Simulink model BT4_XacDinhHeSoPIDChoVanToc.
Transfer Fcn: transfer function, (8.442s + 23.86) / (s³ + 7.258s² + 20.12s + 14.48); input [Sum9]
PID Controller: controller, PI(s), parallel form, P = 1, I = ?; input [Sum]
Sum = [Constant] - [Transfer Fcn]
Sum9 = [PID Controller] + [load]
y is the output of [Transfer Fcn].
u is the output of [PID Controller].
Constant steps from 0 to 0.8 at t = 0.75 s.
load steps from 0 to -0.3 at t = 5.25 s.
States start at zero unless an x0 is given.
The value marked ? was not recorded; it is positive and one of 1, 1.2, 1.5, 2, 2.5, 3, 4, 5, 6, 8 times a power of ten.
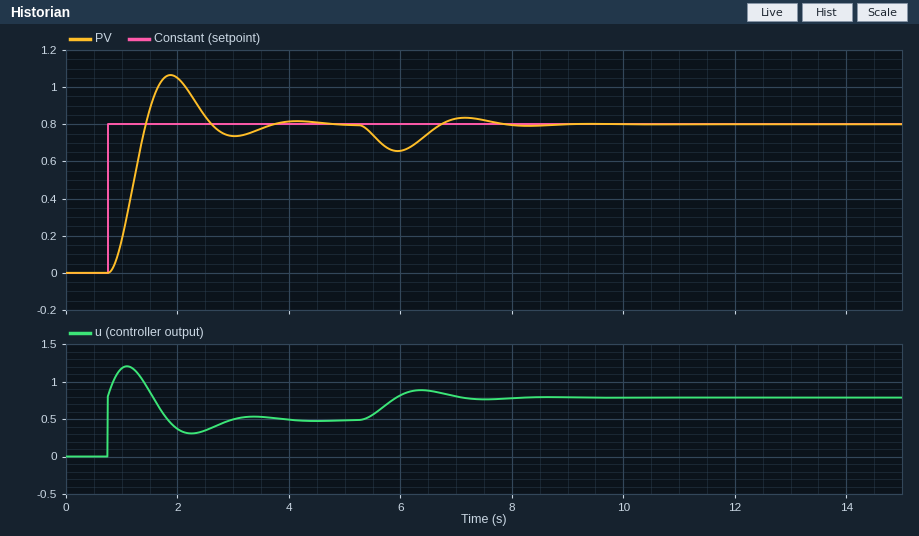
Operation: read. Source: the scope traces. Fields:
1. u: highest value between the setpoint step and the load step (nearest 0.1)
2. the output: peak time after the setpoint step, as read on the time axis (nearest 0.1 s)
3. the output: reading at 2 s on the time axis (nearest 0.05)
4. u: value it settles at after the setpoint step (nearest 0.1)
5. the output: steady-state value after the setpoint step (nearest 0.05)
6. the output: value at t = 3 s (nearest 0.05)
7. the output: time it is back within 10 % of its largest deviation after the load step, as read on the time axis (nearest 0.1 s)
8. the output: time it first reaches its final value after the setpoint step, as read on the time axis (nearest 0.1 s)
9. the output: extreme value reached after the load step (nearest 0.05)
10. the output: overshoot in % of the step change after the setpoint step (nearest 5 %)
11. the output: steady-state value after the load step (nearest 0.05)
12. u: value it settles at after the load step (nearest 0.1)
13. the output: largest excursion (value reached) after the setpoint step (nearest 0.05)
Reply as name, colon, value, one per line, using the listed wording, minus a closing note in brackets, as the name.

u: highest value between the setpoint step and the load step: 1.2
the output: peak time after the setpoint step, as read on the time axis: 1.9 s
the output: reading at 2 s on the time axis: 1.05
u: value it settles at after the setpoint step: 0.5
the output: steady-state value after the setpoint step: 0.80
the output: value at t = 3 s: 0.75
the output: time it is back within 10 % of its largest deviation after the load step, as read on the time axis: 7.6 s
the output: time it first reaches its final value after the setpoint step, as read on the time axis: 1.4 s
the output: extreme value reached after the load step: 0.65
the output: overshoot in % of the step change after the setpoint step: 35 %
the output: steady-state value after the load step: 0.80
u: value it settles at after the load step: 0.8
the output: largest excursion (value reached) after the setpoint step: 1.05
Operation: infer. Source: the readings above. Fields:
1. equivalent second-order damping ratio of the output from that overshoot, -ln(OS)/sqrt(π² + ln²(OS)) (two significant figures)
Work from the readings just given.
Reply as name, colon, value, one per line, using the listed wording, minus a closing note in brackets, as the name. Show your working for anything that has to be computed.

equivalent second-order damping ratio of the output from that overshoot, -ln(OS)/sqrt(π² + ln²(OS)): ln(0.35) = -1.050; 1.050 / sqrt(9.870 + 1.102) = 0.32
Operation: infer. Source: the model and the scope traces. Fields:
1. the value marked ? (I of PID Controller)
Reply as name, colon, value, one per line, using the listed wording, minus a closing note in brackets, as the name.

the value marked ?: 3
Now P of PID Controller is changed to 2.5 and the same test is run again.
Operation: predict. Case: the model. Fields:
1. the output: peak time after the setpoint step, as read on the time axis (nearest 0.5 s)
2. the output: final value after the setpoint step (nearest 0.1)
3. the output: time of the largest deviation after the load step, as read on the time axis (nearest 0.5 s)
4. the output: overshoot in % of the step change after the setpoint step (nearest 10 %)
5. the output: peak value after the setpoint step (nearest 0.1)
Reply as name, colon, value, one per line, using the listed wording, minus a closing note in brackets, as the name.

the output: peak time after the setpoint step, as read on the time axis: 1.5 s
the output: final value after the setpoint step: 0.8
the output: time of the largest deviation after the load step, as read on the time axis: 6.0 s
the output: overshoot in % of the step change after the setpoint step: 20 %
the output: peak value after the setpoint step: 1.0
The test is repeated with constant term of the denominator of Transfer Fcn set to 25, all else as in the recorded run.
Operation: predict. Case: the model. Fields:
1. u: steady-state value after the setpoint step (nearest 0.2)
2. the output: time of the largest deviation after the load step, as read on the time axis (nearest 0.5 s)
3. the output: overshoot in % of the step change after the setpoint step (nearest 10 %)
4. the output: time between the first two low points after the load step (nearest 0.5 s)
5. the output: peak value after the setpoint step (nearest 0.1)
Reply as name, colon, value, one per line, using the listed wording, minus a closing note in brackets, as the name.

u: steady-state value after the setpoint step: 0.8
the output: time of the largest deviation after the load step, as read on the time axis: 6.0 s
the output: overshoot in % of the step change after the setpoint step: 20 %
the output: time between the first two low points after the load step: 2.0 s
the output: peak value after the setpoint step: 1.0
